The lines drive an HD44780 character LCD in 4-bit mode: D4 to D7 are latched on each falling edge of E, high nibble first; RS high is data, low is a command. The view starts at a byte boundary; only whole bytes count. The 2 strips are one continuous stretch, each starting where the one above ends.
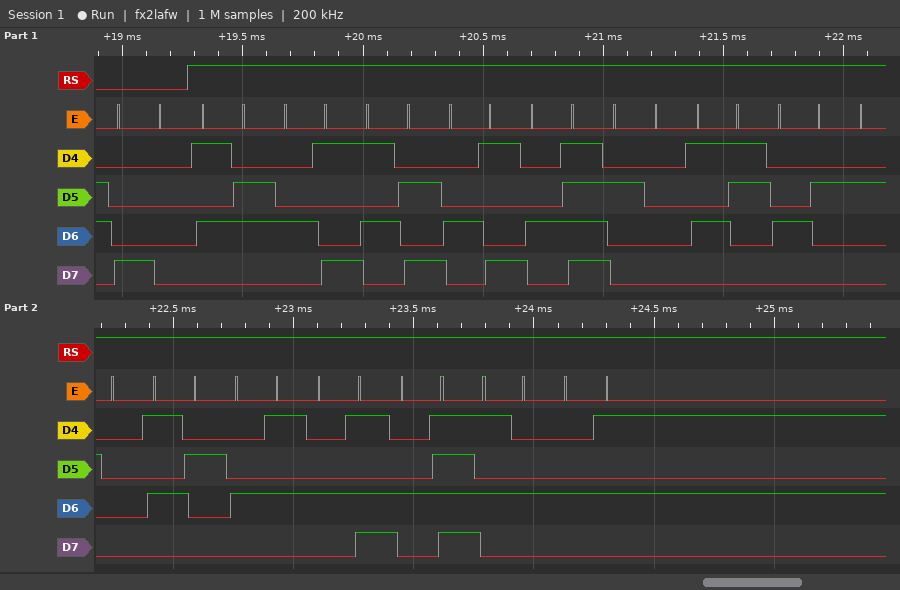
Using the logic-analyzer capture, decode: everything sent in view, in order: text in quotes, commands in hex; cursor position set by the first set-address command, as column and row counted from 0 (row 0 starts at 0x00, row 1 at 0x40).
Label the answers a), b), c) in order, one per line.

a) 0x80 "VIZIO SB REMOTE"
b) column 0, row 0
